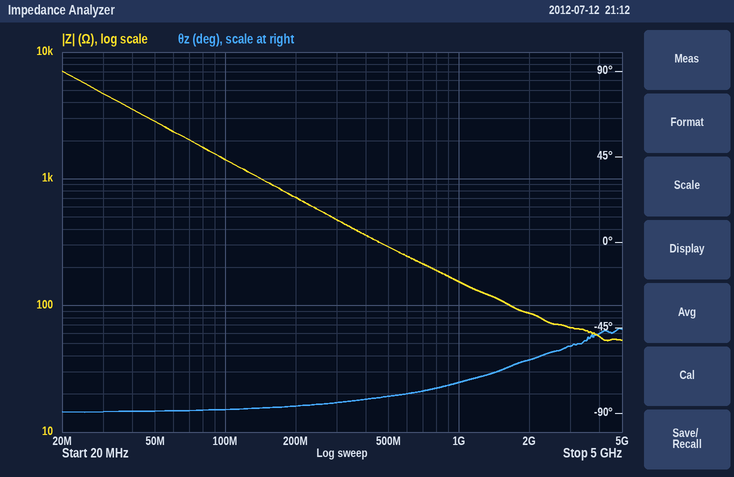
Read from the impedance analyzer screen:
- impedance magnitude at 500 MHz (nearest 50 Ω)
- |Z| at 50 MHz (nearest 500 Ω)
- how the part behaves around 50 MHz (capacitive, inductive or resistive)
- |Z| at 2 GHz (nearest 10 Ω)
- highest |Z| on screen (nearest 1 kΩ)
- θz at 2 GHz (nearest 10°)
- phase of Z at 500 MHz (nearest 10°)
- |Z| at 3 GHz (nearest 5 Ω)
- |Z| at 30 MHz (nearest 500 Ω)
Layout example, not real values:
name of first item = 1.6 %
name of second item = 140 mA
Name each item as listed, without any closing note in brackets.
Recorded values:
impedance magnitude at 500 MHz = 300 Ω
|Z| at 50 MHz = 3.0 kΩ
how the part behaves around 50 MHz = capacitive
|Z| at 2 GHz = 90 Ω
highest |Z| on screen = 7 kΩ
θz at 2 GHz = -60°
phase of Z at 500 MHz = -80°
|Z| at 3 GHz = 65 Ω
|Z| at 30 MHz = 4.5 kΩ
